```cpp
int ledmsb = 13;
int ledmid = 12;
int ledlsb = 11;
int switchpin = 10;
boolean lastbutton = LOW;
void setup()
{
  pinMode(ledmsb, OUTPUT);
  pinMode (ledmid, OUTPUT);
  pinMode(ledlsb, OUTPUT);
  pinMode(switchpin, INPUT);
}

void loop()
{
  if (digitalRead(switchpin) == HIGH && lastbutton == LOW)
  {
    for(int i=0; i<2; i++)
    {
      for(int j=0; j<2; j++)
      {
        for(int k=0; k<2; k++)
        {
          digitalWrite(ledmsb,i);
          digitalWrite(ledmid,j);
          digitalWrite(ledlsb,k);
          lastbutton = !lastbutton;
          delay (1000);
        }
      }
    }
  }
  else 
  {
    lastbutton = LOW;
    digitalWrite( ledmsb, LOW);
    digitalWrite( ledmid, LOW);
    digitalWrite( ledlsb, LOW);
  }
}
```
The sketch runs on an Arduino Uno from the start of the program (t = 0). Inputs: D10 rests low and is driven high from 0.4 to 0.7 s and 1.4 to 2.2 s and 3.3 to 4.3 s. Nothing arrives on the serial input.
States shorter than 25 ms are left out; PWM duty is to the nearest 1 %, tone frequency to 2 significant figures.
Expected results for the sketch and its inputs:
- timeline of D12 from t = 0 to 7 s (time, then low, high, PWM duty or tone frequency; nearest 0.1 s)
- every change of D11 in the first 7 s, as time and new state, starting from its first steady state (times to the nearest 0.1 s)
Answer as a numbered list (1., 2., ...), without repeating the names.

1. 0 s low; 2.4 s high; 4.4 s low; 6.4 s high
2. 0 s low; 1.4 s high; 2.4 s low; 3.4 s high; 4.4 s low; 5.4 s high; 6.4 s low
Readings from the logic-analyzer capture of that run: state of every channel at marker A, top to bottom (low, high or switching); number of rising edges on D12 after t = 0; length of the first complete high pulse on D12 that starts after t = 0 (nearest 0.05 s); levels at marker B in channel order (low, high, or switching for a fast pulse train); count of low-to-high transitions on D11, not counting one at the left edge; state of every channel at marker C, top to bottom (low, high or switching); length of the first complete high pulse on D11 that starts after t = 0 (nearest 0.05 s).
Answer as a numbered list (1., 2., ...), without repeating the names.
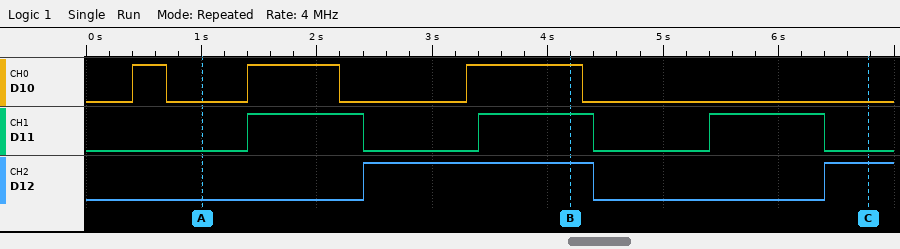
1. D10 low, D11 low, D12 low
2. 2
3. 2.00 s
4. D10 high, D11 high, D12 high
5. 3
6. D10 low, D11 low, D12 high
7. 1.00 s
